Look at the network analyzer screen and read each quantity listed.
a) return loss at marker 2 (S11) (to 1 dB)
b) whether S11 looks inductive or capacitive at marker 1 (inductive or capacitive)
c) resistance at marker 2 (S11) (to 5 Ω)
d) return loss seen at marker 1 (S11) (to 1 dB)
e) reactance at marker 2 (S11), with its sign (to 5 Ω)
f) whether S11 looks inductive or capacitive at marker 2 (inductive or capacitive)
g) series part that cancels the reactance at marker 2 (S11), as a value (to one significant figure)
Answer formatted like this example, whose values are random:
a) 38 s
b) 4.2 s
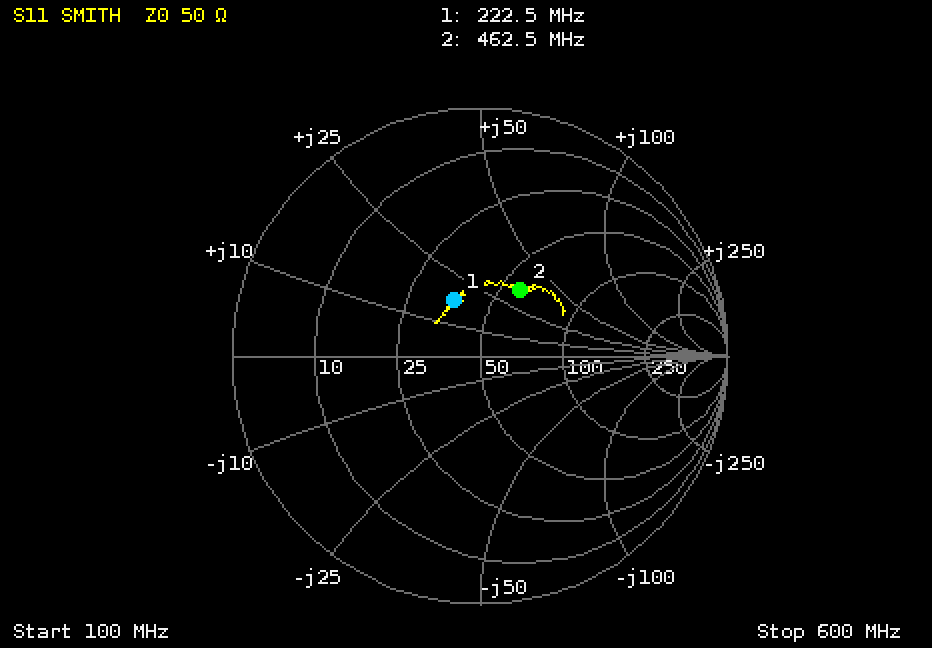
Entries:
a) 10 dB
b) inductive
c) 60 Ω
d) 12 dB
e) +35 Ω
f) inductive
g) 10 pF
